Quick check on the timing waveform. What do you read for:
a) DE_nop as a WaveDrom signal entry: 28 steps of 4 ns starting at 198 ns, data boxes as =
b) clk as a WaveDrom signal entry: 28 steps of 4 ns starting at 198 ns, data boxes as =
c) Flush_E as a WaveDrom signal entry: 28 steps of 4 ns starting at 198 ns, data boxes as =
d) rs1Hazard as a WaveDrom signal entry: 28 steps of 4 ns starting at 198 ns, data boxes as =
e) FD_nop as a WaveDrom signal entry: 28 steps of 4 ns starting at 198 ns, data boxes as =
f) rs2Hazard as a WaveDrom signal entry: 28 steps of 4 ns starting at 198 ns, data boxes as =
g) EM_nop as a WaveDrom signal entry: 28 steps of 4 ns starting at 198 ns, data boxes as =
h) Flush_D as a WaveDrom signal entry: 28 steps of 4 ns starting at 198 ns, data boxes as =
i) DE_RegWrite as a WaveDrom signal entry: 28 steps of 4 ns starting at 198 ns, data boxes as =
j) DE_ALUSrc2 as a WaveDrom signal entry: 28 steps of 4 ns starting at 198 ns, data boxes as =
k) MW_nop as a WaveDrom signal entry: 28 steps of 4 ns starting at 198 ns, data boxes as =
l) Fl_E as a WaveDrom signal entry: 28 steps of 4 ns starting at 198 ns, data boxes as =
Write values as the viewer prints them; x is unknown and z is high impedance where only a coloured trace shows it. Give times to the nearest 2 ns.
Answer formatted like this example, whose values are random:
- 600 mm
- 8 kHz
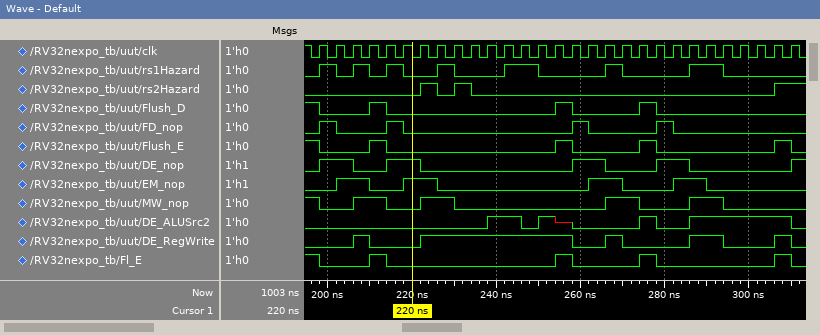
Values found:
- {name: 'DE_nop', wave: '1.0.1.0........1.0..1.0.....'}
- {name: 'clk', wave: 'p...........................'}
- {name: 'Flush_E', wave: '0..10.........10...10......1'}
- {name: 'rs1Hazard', wave: '101010.10..1.0...10...1.0...'}
- {name: 'FD_nop', wave: '10..10.........10...10......'}
- {name: 'rs2Hazard', wave: '0.....1010.................1'}
- {name: 'EM_nop', wave: '01.0.1.0........1.0..1.0....'}
- {name: 'Flush_D', wave: '0..10.........10...10.......'}
- {name: 'DE_RegWrite', wave: '0.10..1........0.10...1.0..1'}
- {name: 'DE_ALUSrc2', wave: '0.........1.01x0...10.1.....'}
- {name: 'MW_nop', wave: '0.1.0.1.0........1.0..1.0...'}
- {name: 'Fl_E', wave: '0..10.........10...10......1'}
